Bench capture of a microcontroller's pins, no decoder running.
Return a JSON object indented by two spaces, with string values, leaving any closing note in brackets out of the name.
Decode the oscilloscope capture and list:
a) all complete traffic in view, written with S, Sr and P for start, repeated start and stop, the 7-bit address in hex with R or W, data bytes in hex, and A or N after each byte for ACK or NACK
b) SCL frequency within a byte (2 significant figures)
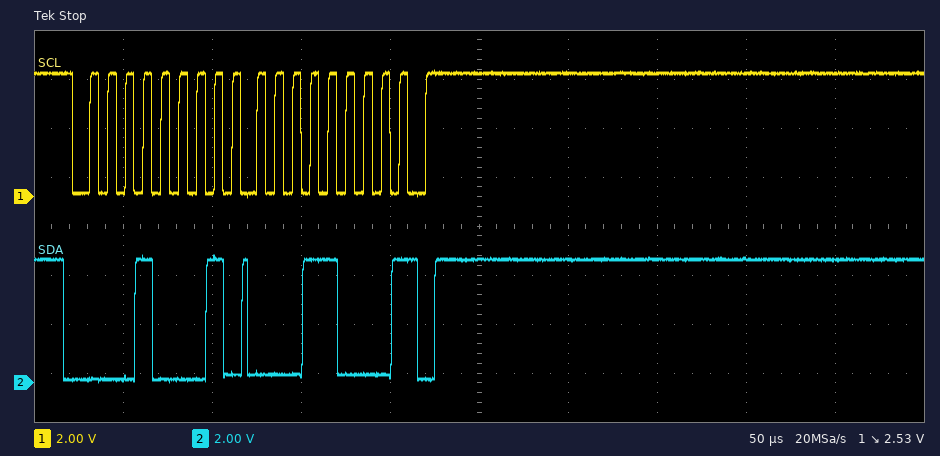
{
  "all complete traffic in view, written with S, Sr and P for start, repeated start and stop, the 7-bit address in hex with R or W, data bytes in hex, and A or N after each byte for ACK or NACK": "S 08R A 18 N P",
  "SCL frequency within a byte": "100 kHz"
}
